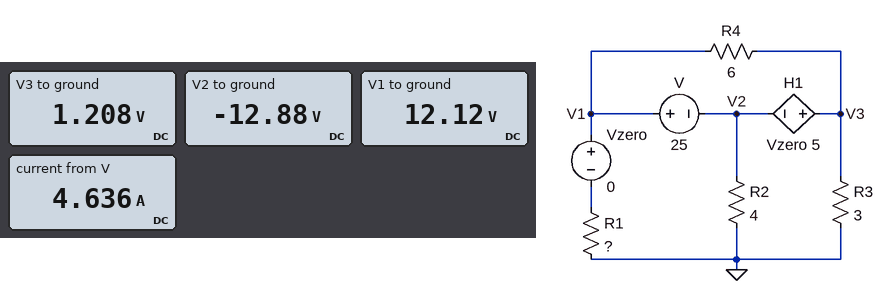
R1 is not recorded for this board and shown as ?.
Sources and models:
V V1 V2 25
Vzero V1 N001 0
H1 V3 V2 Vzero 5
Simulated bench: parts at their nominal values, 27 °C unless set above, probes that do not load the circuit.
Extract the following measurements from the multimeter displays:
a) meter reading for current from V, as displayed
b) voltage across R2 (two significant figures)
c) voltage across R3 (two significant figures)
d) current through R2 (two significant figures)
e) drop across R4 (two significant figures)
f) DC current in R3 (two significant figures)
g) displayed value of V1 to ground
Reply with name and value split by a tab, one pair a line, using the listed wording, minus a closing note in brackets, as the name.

meter reading for current from V, as displayed	4.636 A
voltage across R2	13 V
voltage across R3	1.2 V
current through R2	3.2 A
drop across R4	11 V
DC current in R3	400 mA
displayed value of V1 to ground	12.12 V
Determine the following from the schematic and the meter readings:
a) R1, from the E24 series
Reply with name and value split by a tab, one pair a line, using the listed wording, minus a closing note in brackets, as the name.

R1, from the E24 series	4.3 Ω
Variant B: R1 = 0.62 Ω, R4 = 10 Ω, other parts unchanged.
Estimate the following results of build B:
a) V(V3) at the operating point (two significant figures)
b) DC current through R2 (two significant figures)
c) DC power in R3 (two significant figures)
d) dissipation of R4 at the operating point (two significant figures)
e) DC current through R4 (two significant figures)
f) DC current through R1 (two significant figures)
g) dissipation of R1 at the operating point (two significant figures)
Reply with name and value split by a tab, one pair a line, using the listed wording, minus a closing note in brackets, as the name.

V(V3) at the operating point	2.1 V
DC current through R2	5.5 A
DC power in R3	1.4 W
dissipation of R4 at the operating point	85 mW
DC current through R4	92 mA
DC current through R1	4.8 A
dissipation of R1 at the operating point	14 W
